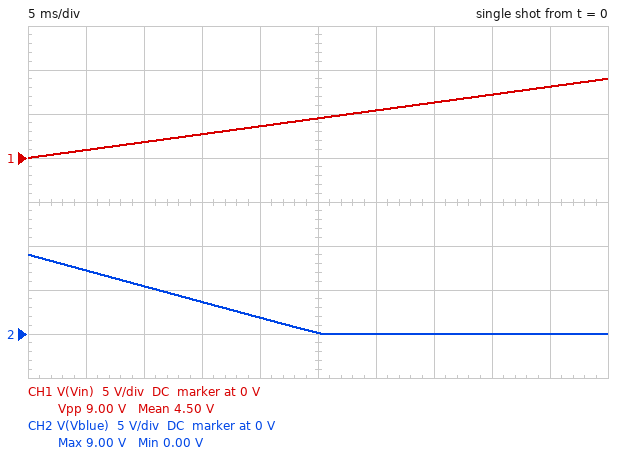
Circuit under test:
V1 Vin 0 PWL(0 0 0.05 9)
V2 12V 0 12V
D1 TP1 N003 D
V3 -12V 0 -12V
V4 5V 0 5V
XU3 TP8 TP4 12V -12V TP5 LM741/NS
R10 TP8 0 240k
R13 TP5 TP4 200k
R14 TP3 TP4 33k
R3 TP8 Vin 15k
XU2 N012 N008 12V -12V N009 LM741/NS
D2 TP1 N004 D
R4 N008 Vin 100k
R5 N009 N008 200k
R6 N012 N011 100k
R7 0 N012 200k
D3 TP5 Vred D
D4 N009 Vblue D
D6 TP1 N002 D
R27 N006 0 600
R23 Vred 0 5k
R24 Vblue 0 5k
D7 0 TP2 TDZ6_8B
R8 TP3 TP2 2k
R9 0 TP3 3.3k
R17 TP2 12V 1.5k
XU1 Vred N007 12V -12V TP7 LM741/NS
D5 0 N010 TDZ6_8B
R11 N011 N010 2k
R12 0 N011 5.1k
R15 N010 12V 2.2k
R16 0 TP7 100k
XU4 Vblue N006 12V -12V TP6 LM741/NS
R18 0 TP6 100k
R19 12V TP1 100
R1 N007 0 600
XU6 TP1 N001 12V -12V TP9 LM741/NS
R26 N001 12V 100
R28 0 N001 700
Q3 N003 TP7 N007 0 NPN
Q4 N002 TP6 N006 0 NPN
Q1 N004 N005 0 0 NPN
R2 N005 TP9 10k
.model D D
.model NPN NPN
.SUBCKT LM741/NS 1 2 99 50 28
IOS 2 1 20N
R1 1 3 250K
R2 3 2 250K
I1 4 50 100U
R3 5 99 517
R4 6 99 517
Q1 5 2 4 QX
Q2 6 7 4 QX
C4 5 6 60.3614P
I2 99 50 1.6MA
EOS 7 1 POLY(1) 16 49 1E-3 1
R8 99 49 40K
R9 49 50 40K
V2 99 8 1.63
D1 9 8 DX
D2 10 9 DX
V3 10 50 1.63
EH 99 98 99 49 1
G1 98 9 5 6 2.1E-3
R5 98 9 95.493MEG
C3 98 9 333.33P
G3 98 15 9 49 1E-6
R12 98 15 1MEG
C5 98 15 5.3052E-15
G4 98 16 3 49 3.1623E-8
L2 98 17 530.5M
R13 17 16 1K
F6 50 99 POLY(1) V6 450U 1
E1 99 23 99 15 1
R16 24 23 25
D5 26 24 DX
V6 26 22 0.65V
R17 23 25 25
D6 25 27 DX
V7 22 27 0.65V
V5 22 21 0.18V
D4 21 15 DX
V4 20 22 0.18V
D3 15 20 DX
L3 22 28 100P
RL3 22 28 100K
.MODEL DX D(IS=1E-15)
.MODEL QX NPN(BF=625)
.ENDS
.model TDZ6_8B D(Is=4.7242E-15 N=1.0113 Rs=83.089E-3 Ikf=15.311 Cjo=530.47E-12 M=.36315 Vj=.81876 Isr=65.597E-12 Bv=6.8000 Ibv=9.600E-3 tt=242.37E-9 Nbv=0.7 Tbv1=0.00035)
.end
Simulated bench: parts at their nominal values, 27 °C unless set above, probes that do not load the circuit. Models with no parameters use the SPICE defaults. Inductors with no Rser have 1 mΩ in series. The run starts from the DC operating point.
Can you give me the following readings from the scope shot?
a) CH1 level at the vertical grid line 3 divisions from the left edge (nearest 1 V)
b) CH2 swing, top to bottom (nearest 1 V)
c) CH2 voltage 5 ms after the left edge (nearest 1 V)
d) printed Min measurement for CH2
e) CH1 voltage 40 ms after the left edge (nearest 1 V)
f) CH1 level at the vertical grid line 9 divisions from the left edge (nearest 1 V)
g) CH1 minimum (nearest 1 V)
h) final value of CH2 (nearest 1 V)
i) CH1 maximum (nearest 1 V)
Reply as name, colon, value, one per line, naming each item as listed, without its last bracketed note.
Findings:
CH1 level at the vertical grid line 3 divisions from the left edge: 3 V
CH2 swing, top to bottom: 9 V
CH2 voltage 5 ms after the left edge: 7 V
printed Min measurement for CH2: 0.00 V
CH1 voltage 40 ms after the left edge: 7 V
CH1 level at the vertical grid line 9 divisions from the left edge: 8 V
CH1 minimum: 0 V
final value of CH2: 0 V
CH1 maximum: 9 V
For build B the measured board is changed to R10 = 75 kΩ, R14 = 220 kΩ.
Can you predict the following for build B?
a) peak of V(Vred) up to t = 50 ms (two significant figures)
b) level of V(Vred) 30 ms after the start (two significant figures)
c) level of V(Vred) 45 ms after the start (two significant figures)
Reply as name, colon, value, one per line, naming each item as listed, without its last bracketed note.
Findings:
peak of V(Vred) up to t = 50 ms: 9.8 V
level of V(Vred) 30 ms after the start: 4.1 V
level of V(Vred) 45 ms after the start: 8.4 V
